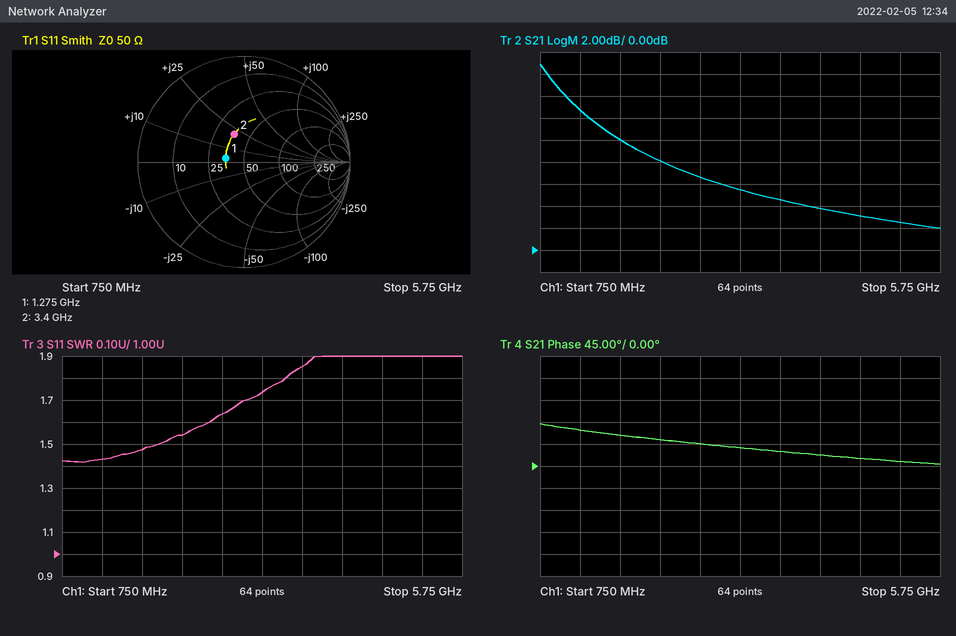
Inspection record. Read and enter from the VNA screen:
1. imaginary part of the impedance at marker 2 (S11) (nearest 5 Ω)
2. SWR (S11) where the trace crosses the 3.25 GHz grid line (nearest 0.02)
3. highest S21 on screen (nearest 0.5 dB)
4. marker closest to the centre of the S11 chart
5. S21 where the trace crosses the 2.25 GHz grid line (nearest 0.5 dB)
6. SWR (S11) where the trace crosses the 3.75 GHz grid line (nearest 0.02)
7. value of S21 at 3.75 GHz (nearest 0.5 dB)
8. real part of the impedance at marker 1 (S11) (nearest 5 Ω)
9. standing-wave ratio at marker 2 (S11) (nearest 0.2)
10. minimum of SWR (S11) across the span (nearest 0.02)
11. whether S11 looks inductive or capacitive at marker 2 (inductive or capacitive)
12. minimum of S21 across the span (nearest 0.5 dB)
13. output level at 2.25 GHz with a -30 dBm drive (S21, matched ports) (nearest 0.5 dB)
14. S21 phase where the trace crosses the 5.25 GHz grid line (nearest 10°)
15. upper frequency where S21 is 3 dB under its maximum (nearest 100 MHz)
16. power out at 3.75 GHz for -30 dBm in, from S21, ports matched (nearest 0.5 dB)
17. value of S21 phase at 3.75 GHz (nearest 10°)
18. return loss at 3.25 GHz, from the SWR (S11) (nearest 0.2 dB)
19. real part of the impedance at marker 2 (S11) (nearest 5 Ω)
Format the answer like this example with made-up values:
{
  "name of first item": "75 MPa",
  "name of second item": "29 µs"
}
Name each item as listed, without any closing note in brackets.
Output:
{
  "imaginary part of the impedance at marker 2 (S11)": "+20 Ω",
  "SWR (S11) where the trace crosses the 3.25 GHz grid line": "1.74",
  "highest S21 on screen": "17.0 dB",
  "marker closest to the centre of the S11 chart": "marker 1",
  "S21 where the trace crosses the 2.25 GHz grid line": "8.0 dB",
  "SWR (S11) where the trace crosses the 3.75 GHz grid line": "1.86",
  "value of S21 at 3.75 GHz": "4.5 dB",
  "real part of the impedance at marker 1 (S11)": "35 Ω",
  "standing-wave ratio at marker 2 (S11)": "1.8",
  "minimum of SWR (S11) across the span": "1.42",
  "whether S11 looks inductive or capacitive at marker 2": "inductive",
  "minimum of S21 across the span": "2.0 dB",
  "output level at 2.25 GHz with a -30 dBm drive (S21, matched ports)": "-22.0 dBm",
  "S21 phase where the trace crosses the 5.25 GHz grid line": "10°",
  "upper frequency where S21 is 3 dB under its maximum": "1.1 GHz",
  "power out at 3.75 GHz for -30 dBm in, from S21, ports matched": "-25.5 dBm",
  "value of S21 phase at 3.75 GHz": "30°",
  "return loss at 3.25 GHz, from the SWR (S11)": "11.4 dB",
  "real part of the impedance at marker 2 (S11)": "35 Ω"
}
